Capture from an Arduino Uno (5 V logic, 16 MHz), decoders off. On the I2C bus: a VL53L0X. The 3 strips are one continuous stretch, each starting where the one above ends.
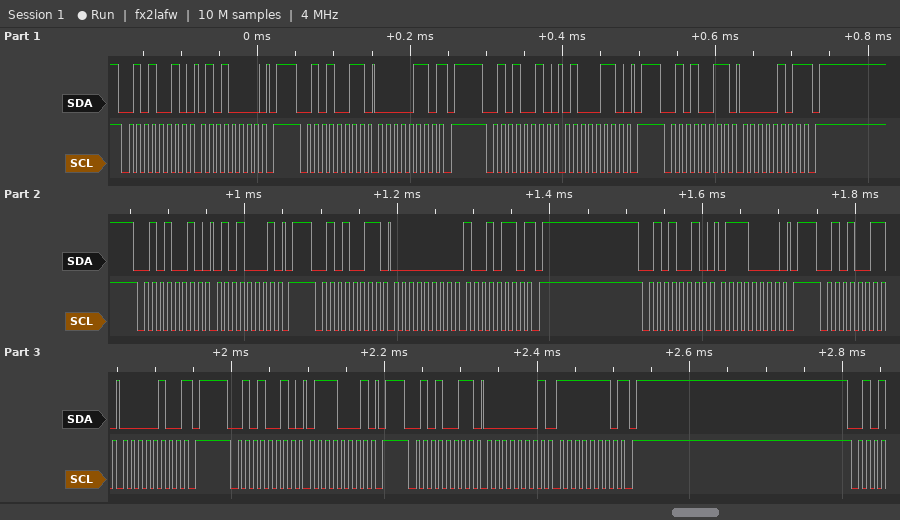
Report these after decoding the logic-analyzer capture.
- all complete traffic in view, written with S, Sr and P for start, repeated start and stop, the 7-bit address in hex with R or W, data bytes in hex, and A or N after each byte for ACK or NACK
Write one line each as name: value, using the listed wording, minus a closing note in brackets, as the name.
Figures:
all complete traffic in view, written with S, Sr and P for start, repeated start and stop, the 7-bit address in hex with R or W, data bytes in hex, and A or N after each byte for ACK or NACK: S 29W A 50 A P S 29R A 06 N P S 29W A 46 A P S 29R A 05 N P S 29W A 51 A P S 29R A 00 A 96 N P S 29W A 70 A P S 29R A 04 N P S 29W A 71 A P S 29R A 01 A FE N P
